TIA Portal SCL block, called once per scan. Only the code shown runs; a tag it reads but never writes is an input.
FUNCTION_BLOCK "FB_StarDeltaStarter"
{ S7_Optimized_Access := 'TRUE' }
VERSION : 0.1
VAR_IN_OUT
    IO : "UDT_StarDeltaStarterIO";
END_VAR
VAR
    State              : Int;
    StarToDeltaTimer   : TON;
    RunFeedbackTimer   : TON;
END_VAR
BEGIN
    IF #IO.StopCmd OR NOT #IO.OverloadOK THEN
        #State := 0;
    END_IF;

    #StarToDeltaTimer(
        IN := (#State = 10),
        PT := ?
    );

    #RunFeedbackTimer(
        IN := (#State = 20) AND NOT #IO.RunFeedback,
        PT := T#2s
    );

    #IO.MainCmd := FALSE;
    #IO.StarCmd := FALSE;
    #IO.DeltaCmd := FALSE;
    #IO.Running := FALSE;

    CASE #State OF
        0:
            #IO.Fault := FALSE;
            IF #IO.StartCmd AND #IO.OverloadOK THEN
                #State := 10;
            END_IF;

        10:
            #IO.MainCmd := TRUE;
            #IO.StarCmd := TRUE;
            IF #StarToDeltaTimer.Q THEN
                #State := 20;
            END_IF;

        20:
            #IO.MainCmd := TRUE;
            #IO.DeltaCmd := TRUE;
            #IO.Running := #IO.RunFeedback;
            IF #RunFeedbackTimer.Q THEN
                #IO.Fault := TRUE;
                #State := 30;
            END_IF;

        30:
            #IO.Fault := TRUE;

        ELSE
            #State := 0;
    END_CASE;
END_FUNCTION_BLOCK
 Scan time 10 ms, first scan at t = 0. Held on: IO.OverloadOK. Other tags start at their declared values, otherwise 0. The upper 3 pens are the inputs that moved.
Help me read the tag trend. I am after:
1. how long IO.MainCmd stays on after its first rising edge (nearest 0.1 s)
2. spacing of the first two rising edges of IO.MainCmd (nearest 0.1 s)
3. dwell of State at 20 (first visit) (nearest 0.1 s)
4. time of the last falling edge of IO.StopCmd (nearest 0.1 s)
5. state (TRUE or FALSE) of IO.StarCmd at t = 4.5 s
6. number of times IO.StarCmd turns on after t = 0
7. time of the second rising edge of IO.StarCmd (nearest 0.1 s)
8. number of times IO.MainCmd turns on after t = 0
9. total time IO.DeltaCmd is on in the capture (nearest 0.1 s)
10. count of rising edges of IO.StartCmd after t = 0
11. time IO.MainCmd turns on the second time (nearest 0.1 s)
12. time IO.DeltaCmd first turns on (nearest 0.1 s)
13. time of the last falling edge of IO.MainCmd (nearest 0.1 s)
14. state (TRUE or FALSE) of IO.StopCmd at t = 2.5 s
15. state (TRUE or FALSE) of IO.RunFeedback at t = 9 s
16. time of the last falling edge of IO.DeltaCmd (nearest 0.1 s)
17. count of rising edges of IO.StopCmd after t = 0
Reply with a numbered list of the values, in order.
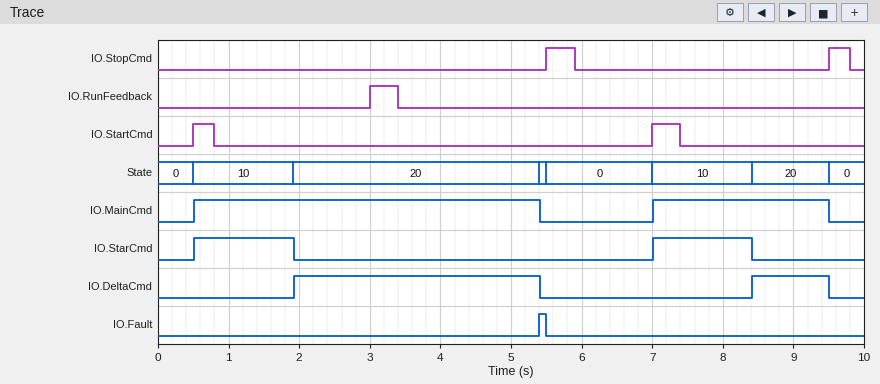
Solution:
1. 4.9 s
2. 6.5 s
3. 3.5 s
4. 9.8 s
5. FALSE
6. 2
7. 7.0 s
8. 2
9. 4.6 s
10. 2
11. 7.0 s
12. 1.9 s
13. 9.5 s
14. FALSE
15. FALSE
16. 9.5 s
17. 2
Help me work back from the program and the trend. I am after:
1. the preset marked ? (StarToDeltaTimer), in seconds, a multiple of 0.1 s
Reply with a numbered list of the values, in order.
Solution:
1. 1.4 s
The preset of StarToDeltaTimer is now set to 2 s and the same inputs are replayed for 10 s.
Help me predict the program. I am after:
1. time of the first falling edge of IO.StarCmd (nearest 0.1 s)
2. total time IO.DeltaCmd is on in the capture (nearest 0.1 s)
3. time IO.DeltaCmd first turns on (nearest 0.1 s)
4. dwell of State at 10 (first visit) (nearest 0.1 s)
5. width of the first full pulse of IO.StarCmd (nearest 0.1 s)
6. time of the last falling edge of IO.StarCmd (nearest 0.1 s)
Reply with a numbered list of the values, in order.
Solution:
1. 2.5 s
2. 3.4 s
3. 2.5 s
4. 2.0 s
5. 2.0 s
6. 9.0 s
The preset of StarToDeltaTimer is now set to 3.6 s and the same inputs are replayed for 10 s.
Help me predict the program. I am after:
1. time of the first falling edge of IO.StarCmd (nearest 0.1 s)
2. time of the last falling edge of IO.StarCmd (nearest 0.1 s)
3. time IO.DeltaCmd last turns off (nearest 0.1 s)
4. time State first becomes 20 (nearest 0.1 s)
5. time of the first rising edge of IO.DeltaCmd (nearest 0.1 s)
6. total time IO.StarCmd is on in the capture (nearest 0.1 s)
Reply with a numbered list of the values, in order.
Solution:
1. 4.1 s
2. 9.5 s
3. 5.5 s
4. 4.1 s
5. 4.1 s
6. 6.1 s
